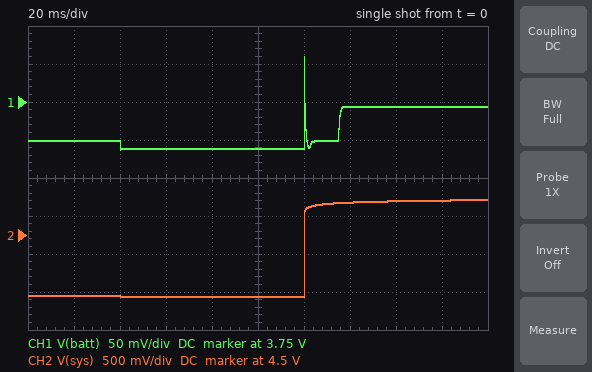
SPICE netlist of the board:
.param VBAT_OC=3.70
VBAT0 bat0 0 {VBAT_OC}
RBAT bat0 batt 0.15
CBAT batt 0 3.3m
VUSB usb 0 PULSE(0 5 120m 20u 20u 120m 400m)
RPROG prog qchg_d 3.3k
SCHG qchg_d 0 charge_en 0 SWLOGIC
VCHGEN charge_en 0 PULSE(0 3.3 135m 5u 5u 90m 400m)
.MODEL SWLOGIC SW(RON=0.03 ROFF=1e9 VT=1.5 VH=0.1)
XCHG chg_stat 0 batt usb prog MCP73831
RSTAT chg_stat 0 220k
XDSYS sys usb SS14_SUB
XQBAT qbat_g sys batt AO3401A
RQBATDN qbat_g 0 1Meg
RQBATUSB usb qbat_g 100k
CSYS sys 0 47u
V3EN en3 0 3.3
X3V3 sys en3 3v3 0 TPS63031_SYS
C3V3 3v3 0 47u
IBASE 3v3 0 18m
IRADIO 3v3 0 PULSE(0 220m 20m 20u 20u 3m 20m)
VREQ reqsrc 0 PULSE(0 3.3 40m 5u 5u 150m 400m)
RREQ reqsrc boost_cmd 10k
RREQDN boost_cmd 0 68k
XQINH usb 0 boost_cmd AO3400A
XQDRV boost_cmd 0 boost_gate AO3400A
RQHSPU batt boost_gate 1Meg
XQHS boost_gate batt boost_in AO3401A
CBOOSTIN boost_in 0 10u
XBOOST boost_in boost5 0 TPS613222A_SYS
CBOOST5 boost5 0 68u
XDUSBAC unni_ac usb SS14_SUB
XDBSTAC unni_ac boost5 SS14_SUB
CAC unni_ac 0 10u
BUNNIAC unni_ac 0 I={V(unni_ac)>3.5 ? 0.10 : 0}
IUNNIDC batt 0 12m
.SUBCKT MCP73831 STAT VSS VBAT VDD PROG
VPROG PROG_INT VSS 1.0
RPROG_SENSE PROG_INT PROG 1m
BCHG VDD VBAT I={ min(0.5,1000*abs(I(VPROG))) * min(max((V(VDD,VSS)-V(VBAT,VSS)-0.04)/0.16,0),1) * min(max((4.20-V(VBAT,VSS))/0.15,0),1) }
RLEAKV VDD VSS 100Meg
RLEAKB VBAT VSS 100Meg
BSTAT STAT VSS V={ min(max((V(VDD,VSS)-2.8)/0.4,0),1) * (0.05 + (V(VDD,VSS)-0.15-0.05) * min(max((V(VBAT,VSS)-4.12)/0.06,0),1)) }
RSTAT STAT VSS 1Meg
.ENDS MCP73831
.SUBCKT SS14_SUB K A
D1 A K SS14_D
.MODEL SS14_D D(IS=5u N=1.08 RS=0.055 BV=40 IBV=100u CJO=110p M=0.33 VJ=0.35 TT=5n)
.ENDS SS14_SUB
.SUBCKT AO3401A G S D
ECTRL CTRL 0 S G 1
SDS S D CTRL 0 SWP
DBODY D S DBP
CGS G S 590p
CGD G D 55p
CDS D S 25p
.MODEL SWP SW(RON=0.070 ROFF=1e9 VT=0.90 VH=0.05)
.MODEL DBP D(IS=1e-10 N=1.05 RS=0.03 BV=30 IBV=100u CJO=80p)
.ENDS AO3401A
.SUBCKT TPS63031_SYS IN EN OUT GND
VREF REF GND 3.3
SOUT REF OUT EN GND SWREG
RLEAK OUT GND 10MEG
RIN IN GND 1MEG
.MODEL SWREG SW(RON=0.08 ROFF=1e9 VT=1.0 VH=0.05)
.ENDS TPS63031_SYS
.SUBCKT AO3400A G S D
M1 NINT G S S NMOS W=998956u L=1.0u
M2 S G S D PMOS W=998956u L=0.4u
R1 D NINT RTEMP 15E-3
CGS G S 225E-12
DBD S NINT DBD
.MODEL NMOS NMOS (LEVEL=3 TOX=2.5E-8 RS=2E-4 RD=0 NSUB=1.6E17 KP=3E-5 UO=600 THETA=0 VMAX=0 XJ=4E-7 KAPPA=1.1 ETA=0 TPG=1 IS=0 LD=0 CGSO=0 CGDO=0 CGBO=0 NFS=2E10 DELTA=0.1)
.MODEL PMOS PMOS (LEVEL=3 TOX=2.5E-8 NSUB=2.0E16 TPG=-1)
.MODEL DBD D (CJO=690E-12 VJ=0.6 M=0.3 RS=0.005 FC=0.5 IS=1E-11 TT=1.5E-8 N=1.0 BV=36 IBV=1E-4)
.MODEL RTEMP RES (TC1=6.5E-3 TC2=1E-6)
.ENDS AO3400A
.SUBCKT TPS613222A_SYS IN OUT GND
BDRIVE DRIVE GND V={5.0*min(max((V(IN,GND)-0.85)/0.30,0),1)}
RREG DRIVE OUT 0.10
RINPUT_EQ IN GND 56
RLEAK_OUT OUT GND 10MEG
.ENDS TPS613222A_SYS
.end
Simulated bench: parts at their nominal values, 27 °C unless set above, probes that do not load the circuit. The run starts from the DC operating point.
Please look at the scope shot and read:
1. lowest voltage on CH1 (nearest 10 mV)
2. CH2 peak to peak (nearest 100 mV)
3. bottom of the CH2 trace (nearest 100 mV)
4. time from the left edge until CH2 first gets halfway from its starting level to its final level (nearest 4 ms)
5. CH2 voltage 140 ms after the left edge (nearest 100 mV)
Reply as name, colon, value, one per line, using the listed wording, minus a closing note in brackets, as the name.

lowest voltage on CH1: 3.69 V
CH2 peak to peak: 1.3 V
bottom of the CH2 trace: 3.7 V
time from the left edge until CH2 first gets halfway from its starting level to its final level: 120 ms
CH2 voltage 140 ms after the left edge: 4.9 V
